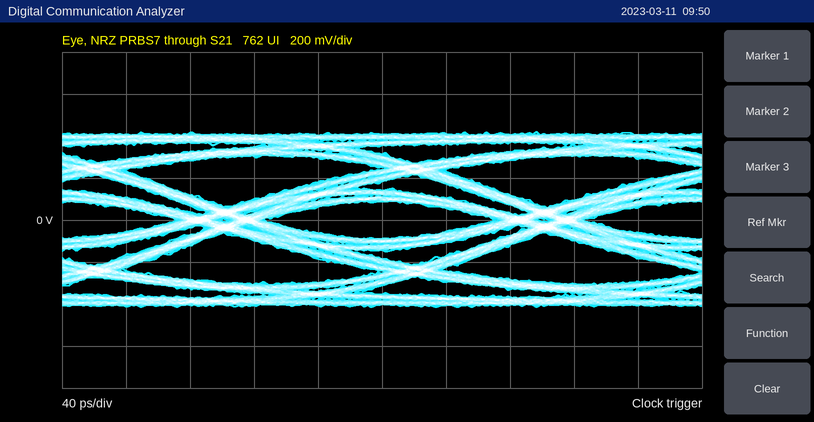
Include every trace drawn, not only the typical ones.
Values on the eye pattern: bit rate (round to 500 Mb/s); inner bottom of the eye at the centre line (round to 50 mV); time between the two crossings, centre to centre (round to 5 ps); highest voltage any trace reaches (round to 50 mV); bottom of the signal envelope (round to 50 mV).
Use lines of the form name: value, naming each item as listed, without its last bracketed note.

bit rate: 5.0 Gb/s
inner bottom of the eye at the centre line: -100 mV
time between the two crossings, centre to centre: 200 ps
highest voltage any trace reaches: 400 mV
bottom of the signal envelope: -400 mV
